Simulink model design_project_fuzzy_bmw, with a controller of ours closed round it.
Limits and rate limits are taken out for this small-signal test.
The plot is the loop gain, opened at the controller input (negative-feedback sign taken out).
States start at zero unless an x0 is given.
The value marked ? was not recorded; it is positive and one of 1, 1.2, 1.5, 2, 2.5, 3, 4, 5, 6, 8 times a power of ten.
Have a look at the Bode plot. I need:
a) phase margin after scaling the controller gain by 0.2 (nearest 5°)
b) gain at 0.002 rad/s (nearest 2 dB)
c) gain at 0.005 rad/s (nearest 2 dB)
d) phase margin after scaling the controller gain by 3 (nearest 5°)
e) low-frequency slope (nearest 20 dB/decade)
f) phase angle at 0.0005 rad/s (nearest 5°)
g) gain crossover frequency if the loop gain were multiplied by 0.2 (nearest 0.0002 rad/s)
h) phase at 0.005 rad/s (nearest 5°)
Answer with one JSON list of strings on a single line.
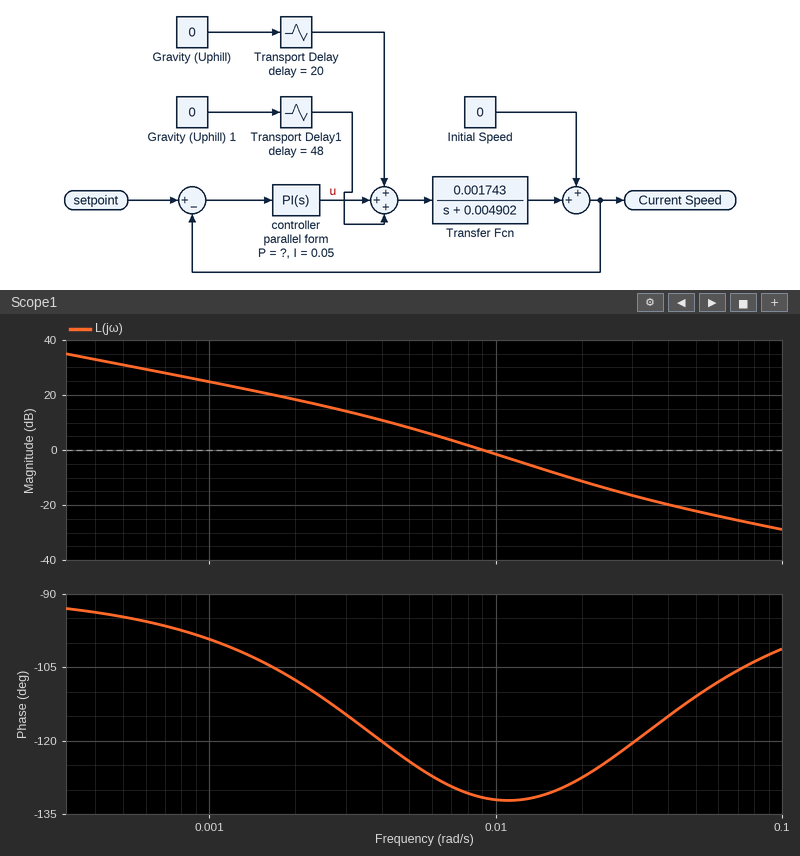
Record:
["65°", "18 dB", "8 dB", "50°", "-20 dB/decade", "-95°", "0.0030 rad/s", "-125°"]
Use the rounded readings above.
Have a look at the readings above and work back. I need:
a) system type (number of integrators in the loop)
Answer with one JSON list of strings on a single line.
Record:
["1"]
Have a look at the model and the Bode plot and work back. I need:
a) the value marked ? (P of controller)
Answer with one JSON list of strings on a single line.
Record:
["2"]
